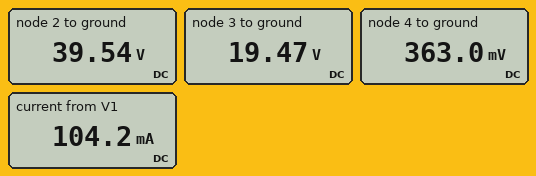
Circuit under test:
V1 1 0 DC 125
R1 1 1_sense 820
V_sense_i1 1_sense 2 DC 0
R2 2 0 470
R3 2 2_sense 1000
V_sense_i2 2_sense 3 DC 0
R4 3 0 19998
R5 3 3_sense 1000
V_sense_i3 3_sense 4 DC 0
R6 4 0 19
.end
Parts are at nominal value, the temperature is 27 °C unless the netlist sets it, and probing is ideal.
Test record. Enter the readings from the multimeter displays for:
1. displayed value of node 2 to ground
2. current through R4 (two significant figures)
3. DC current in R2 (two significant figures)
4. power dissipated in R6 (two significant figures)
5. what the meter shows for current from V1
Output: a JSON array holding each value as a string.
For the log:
["39.54 V", "970 µA", "84 mA", "6.9 mW", "104.2 mA"]
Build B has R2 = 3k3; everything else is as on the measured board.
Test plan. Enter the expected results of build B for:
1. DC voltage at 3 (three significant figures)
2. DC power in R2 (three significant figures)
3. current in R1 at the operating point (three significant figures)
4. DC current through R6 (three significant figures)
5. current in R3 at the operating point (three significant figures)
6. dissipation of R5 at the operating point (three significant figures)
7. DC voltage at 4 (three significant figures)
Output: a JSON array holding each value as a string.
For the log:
["37.0 V", "1.71 W", "60.9 mA", "36.3 mA", "38.1 mA", "1.32 W", "689 mV"]
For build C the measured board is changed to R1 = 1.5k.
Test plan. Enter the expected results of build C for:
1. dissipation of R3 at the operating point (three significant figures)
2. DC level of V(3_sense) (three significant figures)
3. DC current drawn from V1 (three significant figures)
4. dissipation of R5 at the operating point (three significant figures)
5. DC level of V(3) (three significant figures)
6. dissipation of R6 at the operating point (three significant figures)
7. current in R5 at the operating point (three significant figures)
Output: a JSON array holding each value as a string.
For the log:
["164 mW", "232 mV", "66.5 mA", "149 mW", "12.4 V", "2.82 mW", "12.2 mA"]
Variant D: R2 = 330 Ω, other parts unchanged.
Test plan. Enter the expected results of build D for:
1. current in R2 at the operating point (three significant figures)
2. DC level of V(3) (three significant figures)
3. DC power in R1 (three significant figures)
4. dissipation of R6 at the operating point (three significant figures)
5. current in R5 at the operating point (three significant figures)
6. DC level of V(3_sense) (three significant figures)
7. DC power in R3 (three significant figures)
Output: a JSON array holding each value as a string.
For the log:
["97.1 mA", "15.8 V", "10.5 W", "4.55 mW", "15.5 mA", "294 mV", "265 mW"]
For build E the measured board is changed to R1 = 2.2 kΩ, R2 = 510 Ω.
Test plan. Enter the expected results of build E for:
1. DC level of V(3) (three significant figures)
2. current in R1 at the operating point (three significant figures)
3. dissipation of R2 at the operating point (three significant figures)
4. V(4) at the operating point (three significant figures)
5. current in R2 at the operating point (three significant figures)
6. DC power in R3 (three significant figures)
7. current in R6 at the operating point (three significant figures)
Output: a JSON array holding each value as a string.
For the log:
["9.57 V", "48.0 mA", "741 mW", "178 mV", "38.1 mA", "97.4 mW", "9.39 mA"]
